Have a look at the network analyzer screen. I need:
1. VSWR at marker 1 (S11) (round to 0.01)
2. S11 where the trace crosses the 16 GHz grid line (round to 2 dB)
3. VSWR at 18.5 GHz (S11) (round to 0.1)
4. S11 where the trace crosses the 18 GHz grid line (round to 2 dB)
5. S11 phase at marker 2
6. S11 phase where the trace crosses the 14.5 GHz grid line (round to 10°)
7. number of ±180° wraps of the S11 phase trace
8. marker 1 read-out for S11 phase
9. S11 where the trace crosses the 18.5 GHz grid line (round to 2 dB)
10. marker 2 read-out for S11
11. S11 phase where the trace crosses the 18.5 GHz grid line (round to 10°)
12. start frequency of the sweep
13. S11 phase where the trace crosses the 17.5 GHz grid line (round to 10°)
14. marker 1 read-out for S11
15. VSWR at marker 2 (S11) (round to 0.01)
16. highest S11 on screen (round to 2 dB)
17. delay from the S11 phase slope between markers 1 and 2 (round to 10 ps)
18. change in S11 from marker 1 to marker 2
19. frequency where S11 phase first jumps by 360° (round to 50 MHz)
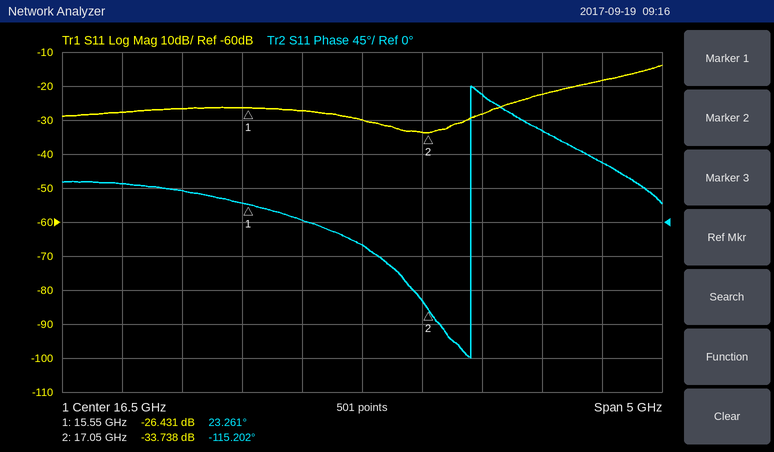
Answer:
1.10
-28 dB
1.3
-22 dB
-115.202°
50°
1
23.261°
-18 dB
-33.738 dB
80°
14 GHz
170°
-26.431 dB
1.04
-14 dB
260 ps
-7.307 dB
17.40 GHz
